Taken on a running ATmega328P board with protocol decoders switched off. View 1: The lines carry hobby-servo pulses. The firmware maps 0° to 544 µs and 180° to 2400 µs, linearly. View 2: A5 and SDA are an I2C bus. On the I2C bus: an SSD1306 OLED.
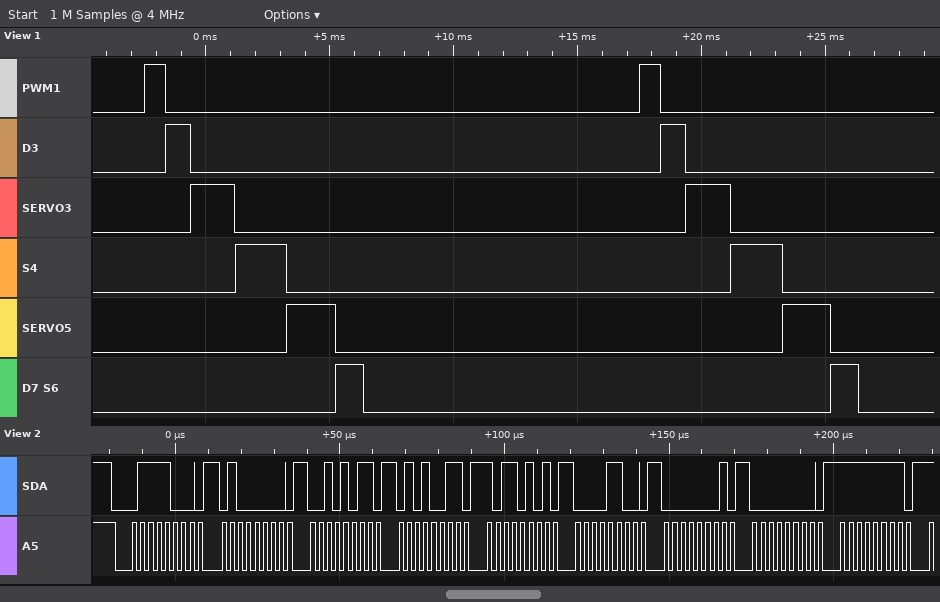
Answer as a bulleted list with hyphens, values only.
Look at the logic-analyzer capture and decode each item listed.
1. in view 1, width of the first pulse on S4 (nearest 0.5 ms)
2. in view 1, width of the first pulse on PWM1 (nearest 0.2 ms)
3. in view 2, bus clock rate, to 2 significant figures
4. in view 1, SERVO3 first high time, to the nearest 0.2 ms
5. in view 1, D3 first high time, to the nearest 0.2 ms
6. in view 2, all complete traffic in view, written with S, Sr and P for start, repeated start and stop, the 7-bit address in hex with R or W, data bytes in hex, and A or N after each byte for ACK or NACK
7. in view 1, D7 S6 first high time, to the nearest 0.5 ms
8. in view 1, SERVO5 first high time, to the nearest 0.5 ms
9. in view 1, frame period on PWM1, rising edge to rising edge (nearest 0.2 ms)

- 2.0 ms
- 0.8 ms
- 400 kHz
- 1.8 ms
- 1.0 ms
- S 3CW A 40 A 2B A 53 A B5 A 0C A 01 A 00 A FF A
- 1.0 ms
- 2.0 ms
- 20.0 ms
